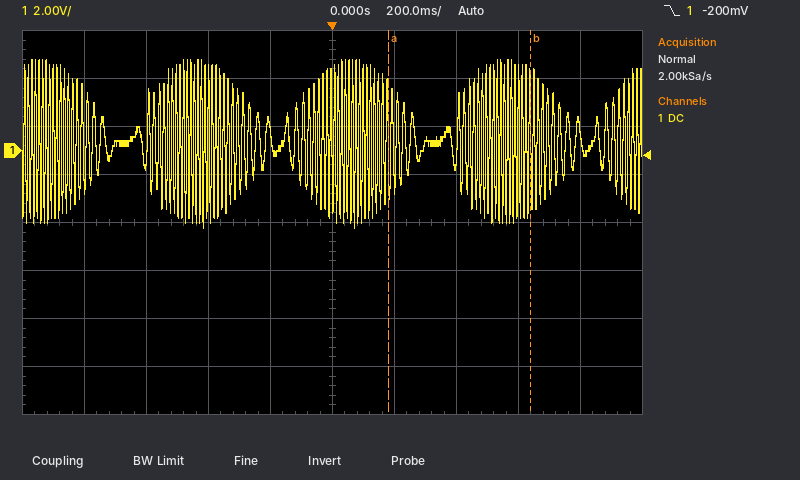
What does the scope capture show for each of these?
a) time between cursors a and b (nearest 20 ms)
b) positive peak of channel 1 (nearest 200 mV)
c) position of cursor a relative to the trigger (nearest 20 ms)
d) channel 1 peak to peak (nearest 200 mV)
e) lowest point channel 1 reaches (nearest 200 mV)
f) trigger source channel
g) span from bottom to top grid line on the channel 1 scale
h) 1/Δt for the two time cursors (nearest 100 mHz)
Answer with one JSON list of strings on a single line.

["460 ms", "3.8 V", "+180 ms", "7.0 V", "-3.2 V", "channel 1", "16 V", "2.2 Hz"]
